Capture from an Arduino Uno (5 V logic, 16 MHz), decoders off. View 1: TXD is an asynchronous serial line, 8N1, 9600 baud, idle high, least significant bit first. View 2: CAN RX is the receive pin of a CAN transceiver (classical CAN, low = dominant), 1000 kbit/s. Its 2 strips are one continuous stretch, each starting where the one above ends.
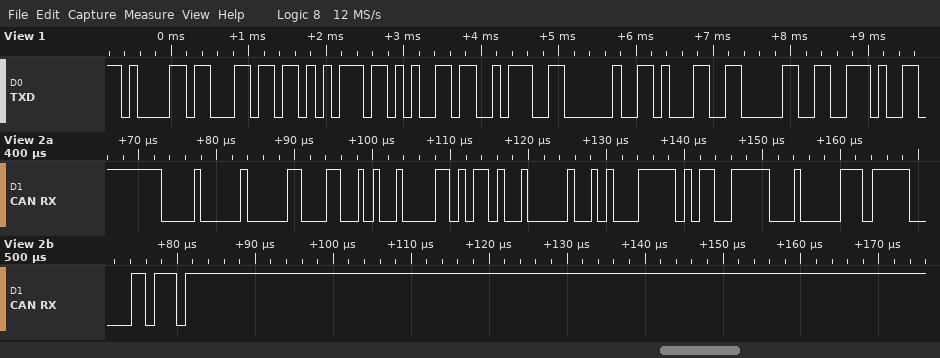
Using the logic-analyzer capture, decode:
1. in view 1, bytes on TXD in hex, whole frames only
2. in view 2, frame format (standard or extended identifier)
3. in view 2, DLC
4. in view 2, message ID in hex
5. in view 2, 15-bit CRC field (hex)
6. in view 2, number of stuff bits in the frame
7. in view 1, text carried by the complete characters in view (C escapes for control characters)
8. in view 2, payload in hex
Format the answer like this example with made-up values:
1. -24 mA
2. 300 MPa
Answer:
1. 61 6C 75 65 3A 20 31 30 2E
2. standard
3. 8
4. 0x080
5. 0x5F0B
6. 8
7. "alue: 10."
8. CA 43 5A 40 51 FB 3E 41
